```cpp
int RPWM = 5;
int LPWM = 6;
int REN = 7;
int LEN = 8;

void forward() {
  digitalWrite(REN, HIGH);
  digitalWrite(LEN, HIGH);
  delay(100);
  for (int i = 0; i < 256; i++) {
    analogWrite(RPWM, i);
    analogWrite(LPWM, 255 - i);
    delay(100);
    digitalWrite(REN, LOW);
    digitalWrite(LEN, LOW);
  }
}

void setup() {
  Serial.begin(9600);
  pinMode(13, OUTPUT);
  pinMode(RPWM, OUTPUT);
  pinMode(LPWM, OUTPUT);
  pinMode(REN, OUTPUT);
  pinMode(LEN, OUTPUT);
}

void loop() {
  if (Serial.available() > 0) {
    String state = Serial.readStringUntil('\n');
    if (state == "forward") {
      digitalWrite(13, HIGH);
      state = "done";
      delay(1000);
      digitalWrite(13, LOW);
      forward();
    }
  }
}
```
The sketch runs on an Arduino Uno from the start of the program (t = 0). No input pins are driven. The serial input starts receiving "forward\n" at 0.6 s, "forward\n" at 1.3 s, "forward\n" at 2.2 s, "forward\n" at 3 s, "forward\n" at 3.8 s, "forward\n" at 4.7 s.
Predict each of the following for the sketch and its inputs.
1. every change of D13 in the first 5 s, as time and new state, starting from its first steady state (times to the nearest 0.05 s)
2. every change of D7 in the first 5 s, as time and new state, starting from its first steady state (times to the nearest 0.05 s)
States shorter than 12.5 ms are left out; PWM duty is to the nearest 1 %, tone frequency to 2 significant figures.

0 s low; 0.6 s high; 1.6 s low
0 s low; 1.6 s high; 1.8 s low
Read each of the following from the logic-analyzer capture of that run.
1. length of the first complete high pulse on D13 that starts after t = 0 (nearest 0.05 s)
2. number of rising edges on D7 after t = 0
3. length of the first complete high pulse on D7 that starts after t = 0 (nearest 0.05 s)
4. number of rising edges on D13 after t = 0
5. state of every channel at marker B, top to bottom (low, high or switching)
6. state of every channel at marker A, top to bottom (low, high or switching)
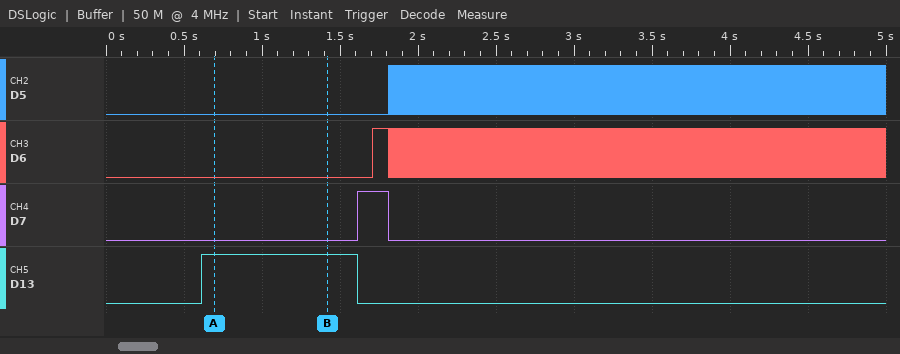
1.00 s
1
0.20 s
1
D5 low, D6 low, D7 low, D13 high
D5 low, D6 low, D7 low, D13 high
